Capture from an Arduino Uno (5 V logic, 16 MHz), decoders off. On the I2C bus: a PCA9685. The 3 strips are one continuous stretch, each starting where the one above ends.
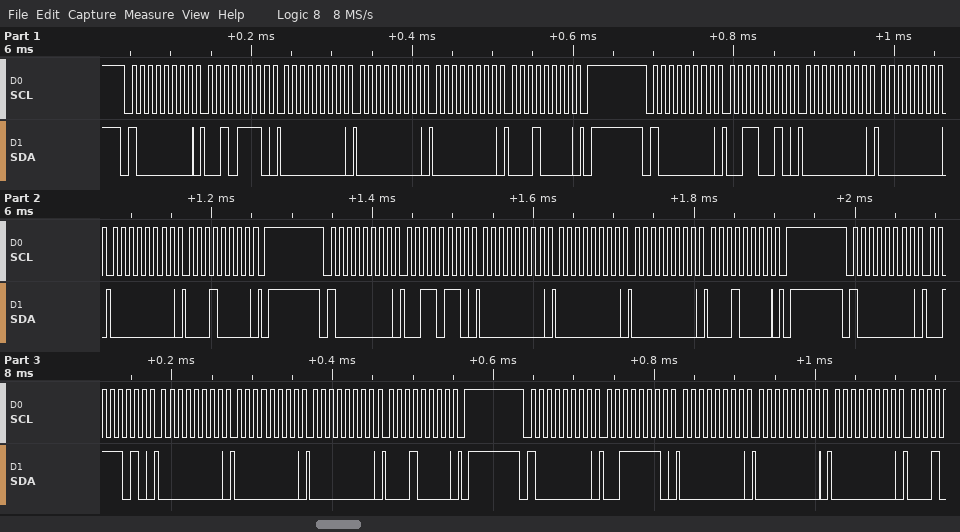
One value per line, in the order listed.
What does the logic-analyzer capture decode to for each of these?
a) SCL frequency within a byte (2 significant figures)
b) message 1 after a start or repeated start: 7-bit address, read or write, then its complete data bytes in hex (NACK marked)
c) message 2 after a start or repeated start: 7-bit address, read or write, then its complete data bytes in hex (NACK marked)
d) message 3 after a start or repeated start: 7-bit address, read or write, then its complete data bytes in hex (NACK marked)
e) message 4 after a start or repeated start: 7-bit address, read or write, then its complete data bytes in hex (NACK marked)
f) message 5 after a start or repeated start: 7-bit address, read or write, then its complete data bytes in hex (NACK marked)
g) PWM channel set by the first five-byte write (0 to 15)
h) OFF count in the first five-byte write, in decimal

100 kHz
0x40 write: 2E 00 00 00 10
0x40 write: 32 00 00 00 10
0x40 write: 36 00 00 00 10
0x40 write: 3A 00 00 00 10
0x40 write: 3E 00 00 00
10
4096
